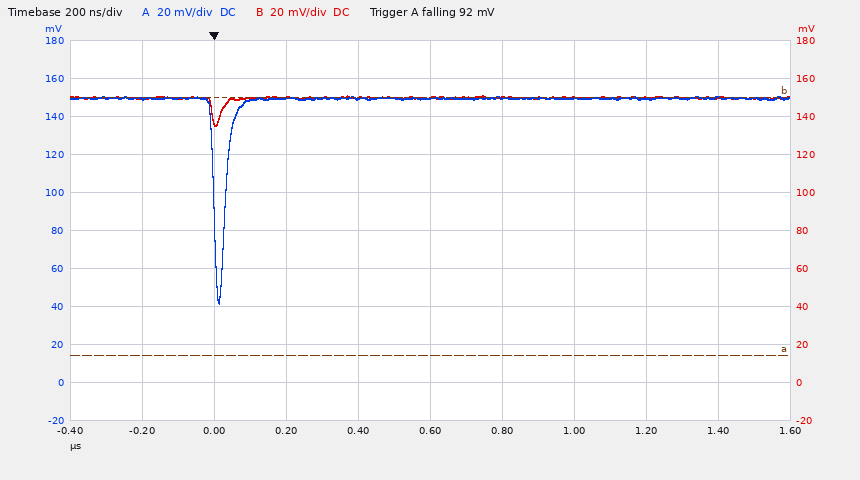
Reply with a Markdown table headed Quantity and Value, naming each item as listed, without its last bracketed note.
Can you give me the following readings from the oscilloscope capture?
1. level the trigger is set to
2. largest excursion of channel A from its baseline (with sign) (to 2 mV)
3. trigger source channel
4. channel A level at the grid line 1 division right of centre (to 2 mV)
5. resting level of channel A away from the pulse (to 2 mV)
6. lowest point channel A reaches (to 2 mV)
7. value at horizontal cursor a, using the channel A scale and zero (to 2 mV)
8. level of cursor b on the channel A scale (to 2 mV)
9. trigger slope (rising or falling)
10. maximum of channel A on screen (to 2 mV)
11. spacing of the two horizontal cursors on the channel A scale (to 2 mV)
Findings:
| Quantity | Value |
|---|---|
| level the trigger is set to | 92 mV |
| largest excursion of channel A from its baseline (with sign) | -108 mV |
| trigger source channel | channel A |
| channel A level at the grid line 1 division right of centre | 150 mV |
| resting level of channel A away from the pulse | 150 mV |
| lowest point channel A reaches | 42 mV |
| value at horizontal cursor a, using the channel A scale and zero | 14 mV |
| level of cursor b on the channel A scale | 150 mV |
| trigger slope | falling |
| maximum of channel A on screen | 150 mV |
| spacing of the two horizontal cursors on the channel A scale | 136 mV |
